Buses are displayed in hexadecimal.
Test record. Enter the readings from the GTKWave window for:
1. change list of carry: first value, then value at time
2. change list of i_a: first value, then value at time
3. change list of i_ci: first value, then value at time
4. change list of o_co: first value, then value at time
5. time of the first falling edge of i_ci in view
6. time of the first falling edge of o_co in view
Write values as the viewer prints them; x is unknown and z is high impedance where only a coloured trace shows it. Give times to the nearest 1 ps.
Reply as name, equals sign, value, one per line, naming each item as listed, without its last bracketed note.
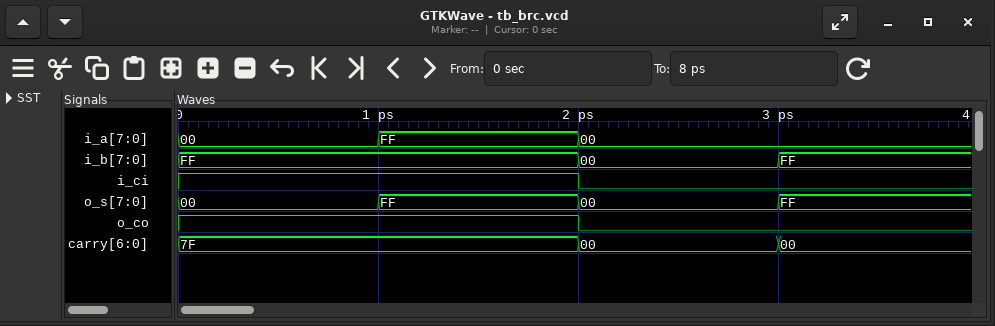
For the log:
change list of carry: first value, then value at time = 7F, 00 at 2 ps
change list of i_a: first value, then value at time = 00, FF at 1 ps, 00 at 2 ps
change list of i_ci: first value, then value at time = 1, 0 at 2 ps
change list of o_co: first value, then value at time = 1, 0 at 2 ps
time of the first falling edge of i_ci in view = 2 ps
time of the first falling edge of o_co in view = 2 ps
